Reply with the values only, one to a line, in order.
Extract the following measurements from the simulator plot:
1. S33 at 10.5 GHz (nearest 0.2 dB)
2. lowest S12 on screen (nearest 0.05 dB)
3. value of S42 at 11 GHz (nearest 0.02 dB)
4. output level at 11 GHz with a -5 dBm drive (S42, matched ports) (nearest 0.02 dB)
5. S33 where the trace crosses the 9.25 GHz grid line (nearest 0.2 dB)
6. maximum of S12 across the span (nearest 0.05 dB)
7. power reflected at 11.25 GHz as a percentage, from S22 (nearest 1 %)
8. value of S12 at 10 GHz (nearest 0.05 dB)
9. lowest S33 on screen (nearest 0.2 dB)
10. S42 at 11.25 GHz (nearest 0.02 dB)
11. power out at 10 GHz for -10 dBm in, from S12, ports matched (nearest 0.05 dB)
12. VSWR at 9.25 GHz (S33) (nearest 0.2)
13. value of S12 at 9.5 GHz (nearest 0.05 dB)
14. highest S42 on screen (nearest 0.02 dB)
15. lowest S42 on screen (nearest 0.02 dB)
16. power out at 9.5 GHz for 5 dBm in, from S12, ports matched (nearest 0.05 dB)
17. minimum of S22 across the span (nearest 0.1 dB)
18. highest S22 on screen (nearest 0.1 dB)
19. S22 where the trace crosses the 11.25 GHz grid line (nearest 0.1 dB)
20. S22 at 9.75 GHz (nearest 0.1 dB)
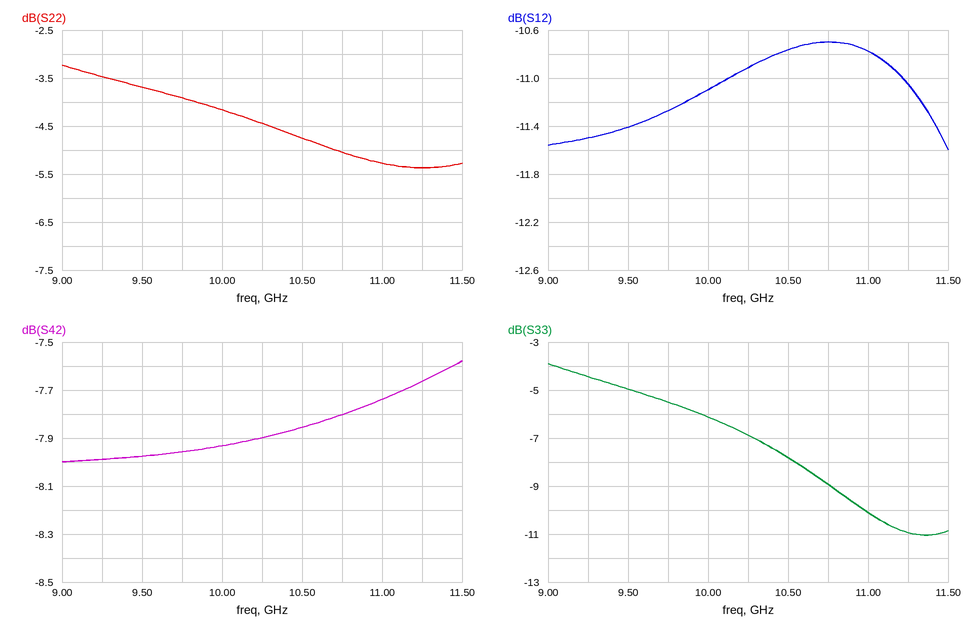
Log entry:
-7.8 dB
-11.60 dB
-7.74 dB
-12.74 dBm
-4.4 dB
-10.70 dB
29 %
-11.10 dB
-11.0 dB
-7.66 dB
-21.10 dBm
4.0
-11.40 dB
-7.58 dB
-8.00 dB
-6.40 dBm
-5.4 dB
-3.2 dB
-5.4 dB
-3.9 dB
